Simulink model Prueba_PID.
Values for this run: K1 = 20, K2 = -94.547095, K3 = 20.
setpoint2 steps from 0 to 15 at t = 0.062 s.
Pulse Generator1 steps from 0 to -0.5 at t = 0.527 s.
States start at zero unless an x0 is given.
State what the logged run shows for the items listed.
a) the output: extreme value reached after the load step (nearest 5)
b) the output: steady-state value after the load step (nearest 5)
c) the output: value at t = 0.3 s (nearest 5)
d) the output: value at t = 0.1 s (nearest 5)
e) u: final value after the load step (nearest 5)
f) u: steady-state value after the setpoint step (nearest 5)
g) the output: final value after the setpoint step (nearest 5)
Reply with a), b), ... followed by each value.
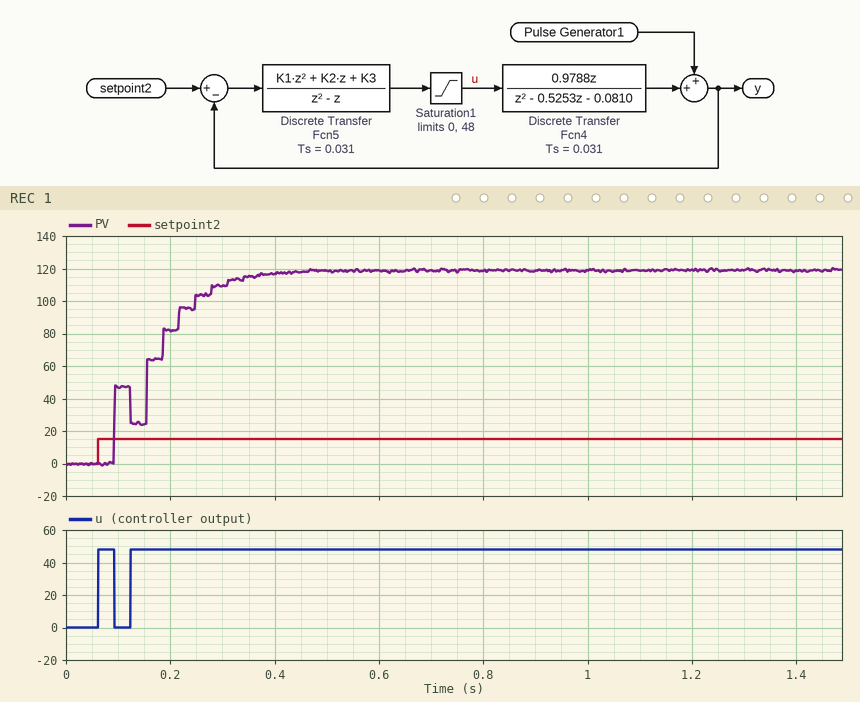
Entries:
a) 120
b) 120
c) 110
d) 45
e) 50
f) 50
g) 120
